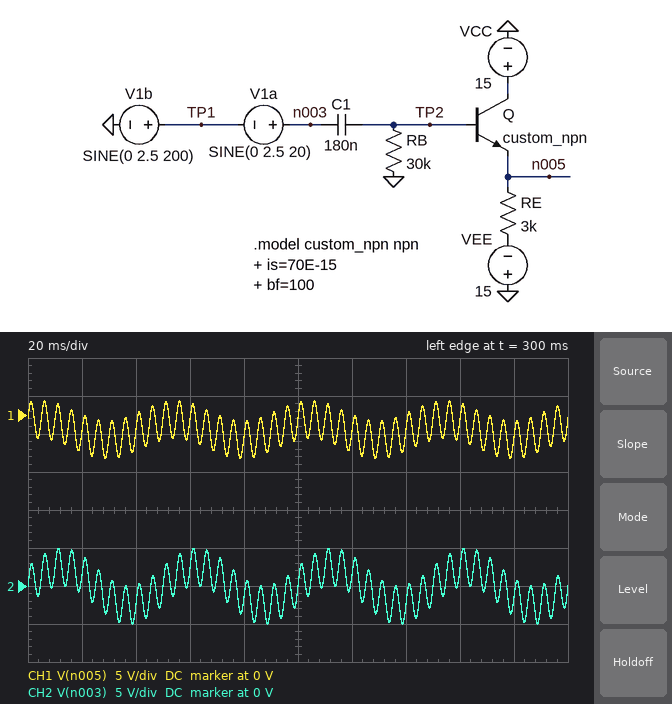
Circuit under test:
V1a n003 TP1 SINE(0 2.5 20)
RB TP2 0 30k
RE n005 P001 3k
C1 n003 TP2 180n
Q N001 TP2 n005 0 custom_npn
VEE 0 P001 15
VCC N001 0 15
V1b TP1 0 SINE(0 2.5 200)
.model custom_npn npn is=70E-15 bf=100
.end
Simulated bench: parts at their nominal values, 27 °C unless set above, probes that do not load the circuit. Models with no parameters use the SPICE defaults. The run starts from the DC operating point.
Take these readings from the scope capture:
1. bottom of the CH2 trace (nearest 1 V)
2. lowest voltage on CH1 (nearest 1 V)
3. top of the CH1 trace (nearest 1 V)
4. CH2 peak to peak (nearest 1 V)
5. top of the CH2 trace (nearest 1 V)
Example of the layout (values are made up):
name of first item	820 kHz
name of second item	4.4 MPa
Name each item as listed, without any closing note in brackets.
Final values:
bottom of the CH2 trace	-5 V
lowest voltage on CH1	-6 V
top of the CH1 trace	2 V
CH2 peak to peak	10 V
top of the CH2 trace	5 V
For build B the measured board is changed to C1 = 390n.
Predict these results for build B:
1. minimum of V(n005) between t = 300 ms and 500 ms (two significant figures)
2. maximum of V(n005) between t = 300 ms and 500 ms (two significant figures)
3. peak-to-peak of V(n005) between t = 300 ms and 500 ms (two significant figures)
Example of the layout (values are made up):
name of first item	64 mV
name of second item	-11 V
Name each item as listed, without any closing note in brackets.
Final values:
minimum of V(n005) between t = 300 ms and 500 ms	-6.4 V
maximum of V(n005) between t = 300 ms and 500 ms	2.5 V
peak-to-peak of V(n005) between t = 300 ms and 500 ms	8.9 V
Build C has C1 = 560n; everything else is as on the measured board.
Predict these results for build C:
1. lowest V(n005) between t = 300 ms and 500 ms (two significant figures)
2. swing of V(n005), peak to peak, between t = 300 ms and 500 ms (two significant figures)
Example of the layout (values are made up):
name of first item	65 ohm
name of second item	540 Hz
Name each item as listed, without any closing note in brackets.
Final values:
lowest V(n005) between t = 300 ms and 500 ms	-6.6 V
swing of V(n005), peak to peak, between t = 300 ms and 500 ms	9.3 V
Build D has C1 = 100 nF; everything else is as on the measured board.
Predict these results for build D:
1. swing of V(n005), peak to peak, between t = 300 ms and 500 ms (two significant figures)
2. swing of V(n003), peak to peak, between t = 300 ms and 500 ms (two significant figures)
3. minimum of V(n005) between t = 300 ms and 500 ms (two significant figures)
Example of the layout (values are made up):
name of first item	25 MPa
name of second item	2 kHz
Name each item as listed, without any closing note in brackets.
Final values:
swing of V(n005), peak to peak, between t = 300 ms and 500 ms	6.4 V
swing of V(n003), peak to peak, between t = 300 ms and 500 ms	9.9 V
minimum of V(n005) between t = 300 ms and 500 ms	-5.1 V
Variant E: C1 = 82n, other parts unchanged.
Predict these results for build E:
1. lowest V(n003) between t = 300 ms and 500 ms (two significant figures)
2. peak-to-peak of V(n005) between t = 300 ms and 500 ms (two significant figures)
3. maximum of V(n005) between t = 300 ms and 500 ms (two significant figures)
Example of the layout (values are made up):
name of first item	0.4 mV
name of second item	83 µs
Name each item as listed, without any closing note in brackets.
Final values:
lowest V(n003) between t = 300 ms and 500 ms	-5.0 V
peak-to-peak of V(n005) between t = 300 ms and 500 ms	6.0 V
maximum of V(n005) between t = 300 ms and 500 ms	1.1 V
